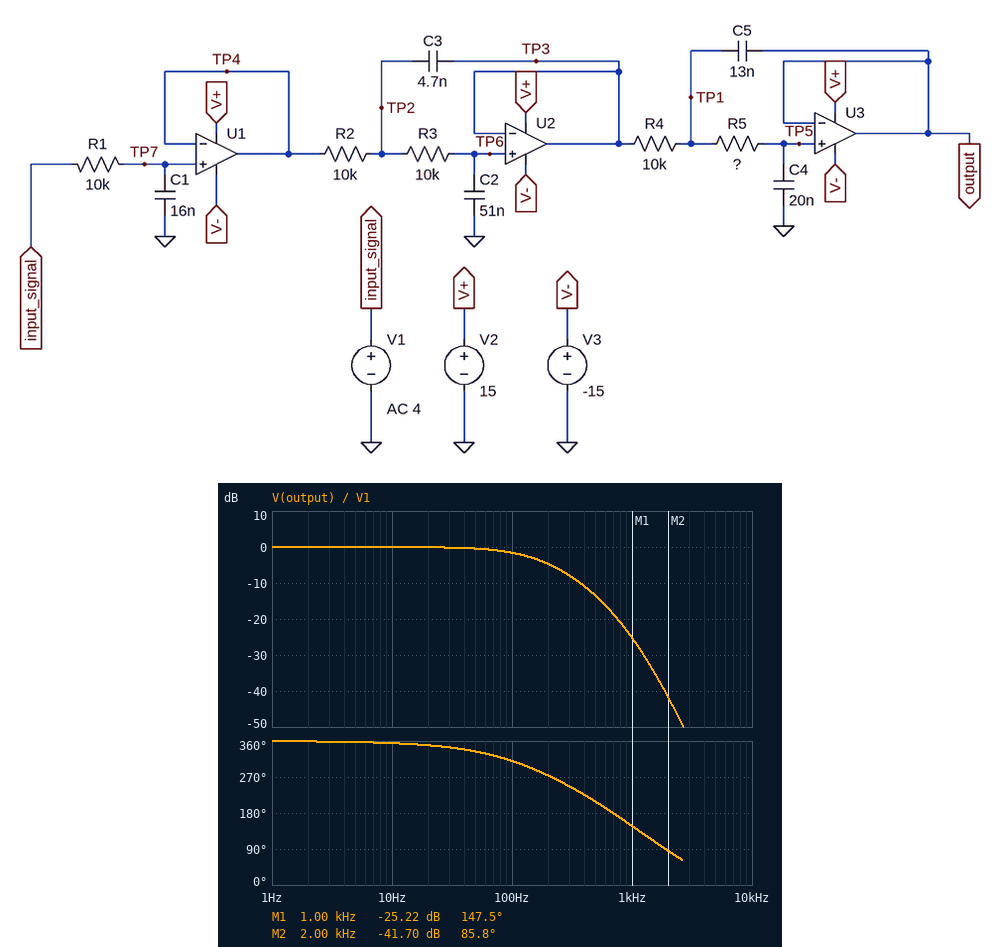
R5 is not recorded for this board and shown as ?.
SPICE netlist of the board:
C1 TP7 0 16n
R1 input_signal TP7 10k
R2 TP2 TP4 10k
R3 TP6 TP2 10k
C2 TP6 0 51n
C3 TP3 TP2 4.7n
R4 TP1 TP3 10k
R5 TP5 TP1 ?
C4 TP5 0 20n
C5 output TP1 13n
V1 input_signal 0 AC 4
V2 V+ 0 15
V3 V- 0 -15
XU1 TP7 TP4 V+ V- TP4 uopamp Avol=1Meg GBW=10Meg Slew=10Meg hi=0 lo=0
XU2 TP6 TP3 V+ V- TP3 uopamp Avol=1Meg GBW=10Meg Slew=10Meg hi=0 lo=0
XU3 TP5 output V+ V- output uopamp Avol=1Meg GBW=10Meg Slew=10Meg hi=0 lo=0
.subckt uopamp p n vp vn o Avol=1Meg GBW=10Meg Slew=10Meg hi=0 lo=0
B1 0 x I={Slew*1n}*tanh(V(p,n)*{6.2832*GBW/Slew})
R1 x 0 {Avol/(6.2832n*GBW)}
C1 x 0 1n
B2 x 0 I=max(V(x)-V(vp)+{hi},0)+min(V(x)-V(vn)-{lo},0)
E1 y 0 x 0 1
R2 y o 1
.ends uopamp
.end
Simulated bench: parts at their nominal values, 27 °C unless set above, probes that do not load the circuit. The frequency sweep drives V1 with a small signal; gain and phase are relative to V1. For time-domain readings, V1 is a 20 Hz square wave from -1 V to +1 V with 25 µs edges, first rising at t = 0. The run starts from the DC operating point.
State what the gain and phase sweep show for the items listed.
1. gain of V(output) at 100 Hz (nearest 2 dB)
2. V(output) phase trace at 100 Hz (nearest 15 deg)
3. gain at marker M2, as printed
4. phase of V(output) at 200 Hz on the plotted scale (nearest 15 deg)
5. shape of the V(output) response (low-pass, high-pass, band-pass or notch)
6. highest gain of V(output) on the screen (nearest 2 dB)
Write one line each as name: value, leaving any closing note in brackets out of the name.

gain of V(output) at 100 Hz: -2 dB
V(output) phase trace at 100 Hz: 315 deg
gain at marker M2, as printed: -41.70 dB
phase of V(output) at 200 Hz on the plotted scale: 270 deg
shape of the V(output) response: low-pass
highest gain of V(output) on the screen: 0 dB
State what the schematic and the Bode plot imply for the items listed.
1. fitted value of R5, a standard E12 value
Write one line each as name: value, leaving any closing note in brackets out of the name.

fitted value of R5, a standard E12 value: 5.6 kΩ
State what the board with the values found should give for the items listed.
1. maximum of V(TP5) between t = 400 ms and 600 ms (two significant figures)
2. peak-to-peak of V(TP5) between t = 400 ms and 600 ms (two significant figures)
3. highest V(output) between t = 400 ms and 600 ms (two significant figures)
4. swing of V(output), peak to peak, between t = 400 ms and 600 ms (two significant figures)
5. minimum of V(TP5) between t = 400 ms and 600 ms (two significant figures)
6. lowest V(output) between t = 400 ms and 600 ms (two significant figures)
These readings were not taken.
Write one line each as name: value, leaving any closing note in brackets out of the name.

maximum of V(TP5) between t = 400 ms and 600 ms: 1.0 V
peak-to-peak of V(TP5) between t = 400 ms and 600 ms: 2.0 V
highest V(output) between t = 400 ms and 600 ms: 1.0 V
swing of V(output), peak to peak, between t = 400 ms and 600 ms: 2.0 V
minimum of V(TP5) between t = 400 ms and 600 ms: -1.0 V
lowest V(output) between t = 400 ms and 600 ms: -1.0 V
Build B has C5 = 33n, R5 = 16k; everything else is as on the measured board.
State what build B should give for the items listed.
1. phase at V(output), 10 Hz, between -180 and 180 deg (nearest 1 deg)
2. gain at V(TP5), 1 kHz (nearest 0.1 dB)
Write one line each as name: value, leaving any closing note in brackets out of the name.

phase at V(output), 10 Hz, between -180 and 180 deg: -6 deg
gain at V(TP5), 1 kHz: -32.3 dB
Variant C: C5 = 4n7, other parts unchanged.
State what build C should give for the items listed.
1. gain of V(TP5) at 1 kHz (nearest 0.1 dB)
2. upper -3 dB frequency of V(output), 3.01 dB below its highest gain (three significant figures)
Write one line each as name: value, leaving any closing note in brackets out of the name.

gain of V(TP5) at 1 kHz: -25.7 dB
upper -3 dB frequency of V(output), 3.01 dB below its highest gain: 145 Hz
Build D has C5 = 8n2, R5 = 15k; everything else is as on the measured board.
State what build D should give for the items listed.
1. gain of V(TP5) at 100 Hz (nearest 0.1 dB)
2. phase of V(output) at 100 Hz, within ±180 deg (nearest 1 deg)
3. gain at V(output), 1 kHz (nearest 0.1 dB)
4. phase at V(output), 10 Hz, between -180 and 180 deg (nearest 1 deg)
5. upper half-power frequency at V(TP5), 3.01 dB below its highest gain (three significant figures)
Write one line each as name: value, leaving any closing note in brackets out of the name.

gain of V(TP5) at 100 Hz: -1.8 dB
phase of V(output) at 100 Hz, within ±180 deg: -56 deg
gain at V(output), 1 kHz: -29.1 dB
phase at V(output), 10 Hz, between -180 and 180 deg: -6 deg
upper half-power frequency at V(TP5), 3.01 dB below its highest gain: 135 Hz
